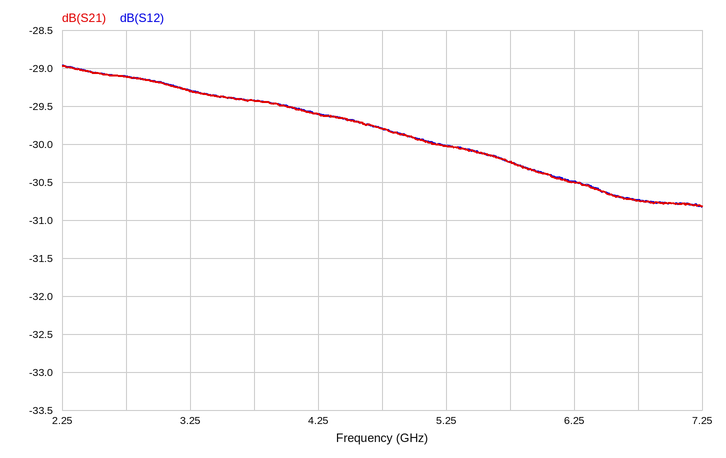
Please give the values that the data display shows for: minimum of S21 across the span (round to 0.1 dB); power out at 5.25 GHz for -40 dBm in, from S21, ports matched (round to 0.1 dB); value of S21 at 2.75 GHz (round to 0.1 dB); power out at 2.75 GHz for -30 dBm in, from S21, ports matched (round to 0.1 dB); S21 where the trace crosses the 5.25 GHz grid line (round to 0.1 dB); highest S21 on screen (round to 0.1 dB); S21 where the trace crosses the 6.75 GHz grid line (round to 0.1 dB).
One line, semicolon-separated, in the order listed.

-30.8 dB; -70.0 dBm; -29.1 dB; -59.1 dBm; -30.0 dB; -29.0 dB; -30.7 dB
